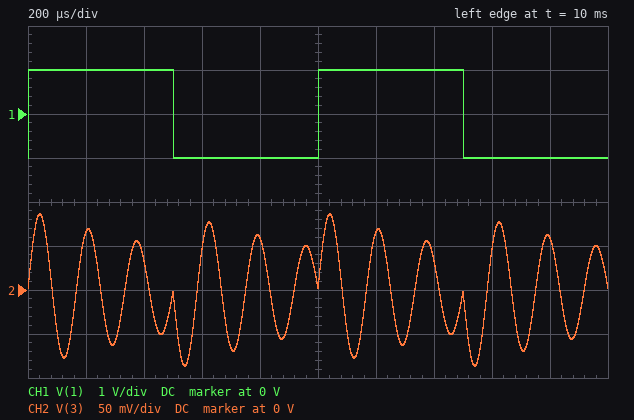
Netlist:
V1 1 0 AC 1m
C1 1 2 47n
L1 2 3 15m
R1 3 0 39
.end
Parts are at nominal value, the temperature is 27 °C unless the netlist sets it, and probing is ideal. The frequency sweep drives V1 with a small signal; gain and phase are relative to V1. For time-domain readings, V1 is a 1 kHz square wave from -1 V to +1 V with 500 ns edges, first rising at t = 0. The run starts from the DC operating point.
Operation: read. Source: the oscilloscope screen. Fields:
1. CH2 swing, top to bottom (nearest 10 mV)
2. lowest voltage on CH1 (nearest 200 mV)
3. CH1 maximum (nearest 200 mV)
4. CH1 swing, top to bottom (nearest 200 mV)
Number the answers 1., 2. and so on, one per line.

1. 170 mV
2. -1.0 V
3. 1.0 V
4. 2.0 V
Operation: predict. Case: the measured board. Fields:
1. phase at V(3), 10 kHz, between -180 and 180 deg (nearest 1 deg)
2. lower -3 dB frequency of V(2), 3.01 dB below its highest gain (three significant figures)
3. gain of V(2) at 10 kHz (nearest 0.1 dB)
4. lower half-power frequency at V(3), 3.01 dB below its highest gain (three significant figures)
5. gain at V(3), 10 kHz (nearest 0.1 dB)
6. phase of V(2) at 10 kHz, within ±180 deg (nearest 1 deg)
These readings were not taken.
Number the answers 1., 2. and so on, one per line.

1. -86 deg
2. 5.80 kHz
3. 3.9 dB
4. 5.79 kHz
5. -23.8 dB
6. 1 deg
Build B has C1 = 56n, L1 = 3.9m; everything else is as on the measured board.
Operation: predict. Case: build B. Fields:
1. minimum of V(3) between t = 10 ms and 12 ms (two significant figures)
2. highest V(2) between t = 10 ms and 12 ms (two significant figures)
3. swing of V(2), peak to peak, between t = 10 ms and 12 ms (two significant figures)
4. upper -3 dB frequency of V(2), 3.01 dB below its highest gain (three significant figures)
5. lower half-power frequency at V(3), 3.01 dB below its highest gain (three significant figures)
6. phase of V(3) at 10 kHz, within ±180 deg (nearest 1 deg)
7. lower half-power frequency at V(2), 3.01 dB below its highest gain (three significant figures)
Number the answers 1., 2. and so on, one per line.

1. -280 mV
2. 2.1 V
3. 4.2 V
4. 11.7 kHz
5. 10.0 kHz
6. 45 deg
7. 10.1 kHz
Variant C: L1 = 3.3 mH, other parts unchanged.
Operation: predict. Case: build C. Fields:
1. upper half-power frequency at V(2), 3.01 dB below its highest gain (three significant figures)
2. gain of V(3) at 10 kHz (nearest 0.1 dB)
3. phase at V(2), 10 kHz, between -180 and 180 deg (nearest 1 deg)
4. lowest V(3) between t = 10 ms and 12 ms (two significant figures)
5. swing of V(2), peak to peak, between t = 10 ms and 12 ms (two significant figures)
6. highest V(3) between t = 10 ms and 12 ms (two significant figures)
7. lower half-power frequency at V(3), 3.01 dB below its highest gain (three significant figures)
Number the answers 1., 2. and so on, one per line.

1. 13.9 kHz
2. -10.9 dB
3. 153 deg
4. -270 mV
5. 4.1 V
6. 270 mV
7. 11.9 kHz
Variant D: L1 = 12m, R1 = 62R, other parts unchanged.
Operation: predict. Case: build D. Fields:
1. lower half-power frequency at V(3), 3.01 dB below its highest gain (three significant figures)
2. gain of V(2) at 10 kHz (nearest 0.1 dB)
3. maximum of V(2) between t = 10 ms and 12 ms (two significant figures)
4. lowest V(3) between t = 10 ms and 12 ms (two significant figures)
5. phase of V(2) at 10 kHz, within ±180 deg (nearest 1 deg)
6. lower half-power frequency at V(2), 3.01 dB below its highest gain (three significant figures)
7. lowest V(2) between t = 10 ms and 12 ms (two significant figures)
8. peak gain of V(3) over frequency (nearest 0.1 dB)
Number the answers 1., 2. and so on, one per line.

1. 6.30 kHz
2. 5.1 dB
3. 2.2 V
4. -250 mV
5. 4 deg
6. 6.35 kHz
7. -2.2 V
8. 0 dB
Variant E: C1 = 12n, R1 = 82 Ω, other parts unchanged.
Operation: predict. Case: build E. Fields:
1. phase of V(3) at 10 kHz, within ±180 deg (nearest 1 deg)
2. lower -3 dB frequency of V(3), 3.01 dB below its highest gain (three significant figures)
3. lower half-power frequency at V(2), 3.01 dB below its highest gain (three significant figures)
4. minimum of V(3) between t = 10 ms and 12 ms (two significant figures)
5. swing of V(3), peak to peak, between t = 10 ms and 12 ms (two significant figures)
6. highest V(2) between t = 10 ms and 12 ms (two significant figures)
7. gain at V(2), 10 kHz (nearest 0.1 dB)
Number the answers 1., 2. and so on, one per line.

1. 78 deg
2. 11.4 kHz
3. 11.5 kHz
4. -110 mV
5. 230 mV
6. 1.6 V
7. 7.6 dB
